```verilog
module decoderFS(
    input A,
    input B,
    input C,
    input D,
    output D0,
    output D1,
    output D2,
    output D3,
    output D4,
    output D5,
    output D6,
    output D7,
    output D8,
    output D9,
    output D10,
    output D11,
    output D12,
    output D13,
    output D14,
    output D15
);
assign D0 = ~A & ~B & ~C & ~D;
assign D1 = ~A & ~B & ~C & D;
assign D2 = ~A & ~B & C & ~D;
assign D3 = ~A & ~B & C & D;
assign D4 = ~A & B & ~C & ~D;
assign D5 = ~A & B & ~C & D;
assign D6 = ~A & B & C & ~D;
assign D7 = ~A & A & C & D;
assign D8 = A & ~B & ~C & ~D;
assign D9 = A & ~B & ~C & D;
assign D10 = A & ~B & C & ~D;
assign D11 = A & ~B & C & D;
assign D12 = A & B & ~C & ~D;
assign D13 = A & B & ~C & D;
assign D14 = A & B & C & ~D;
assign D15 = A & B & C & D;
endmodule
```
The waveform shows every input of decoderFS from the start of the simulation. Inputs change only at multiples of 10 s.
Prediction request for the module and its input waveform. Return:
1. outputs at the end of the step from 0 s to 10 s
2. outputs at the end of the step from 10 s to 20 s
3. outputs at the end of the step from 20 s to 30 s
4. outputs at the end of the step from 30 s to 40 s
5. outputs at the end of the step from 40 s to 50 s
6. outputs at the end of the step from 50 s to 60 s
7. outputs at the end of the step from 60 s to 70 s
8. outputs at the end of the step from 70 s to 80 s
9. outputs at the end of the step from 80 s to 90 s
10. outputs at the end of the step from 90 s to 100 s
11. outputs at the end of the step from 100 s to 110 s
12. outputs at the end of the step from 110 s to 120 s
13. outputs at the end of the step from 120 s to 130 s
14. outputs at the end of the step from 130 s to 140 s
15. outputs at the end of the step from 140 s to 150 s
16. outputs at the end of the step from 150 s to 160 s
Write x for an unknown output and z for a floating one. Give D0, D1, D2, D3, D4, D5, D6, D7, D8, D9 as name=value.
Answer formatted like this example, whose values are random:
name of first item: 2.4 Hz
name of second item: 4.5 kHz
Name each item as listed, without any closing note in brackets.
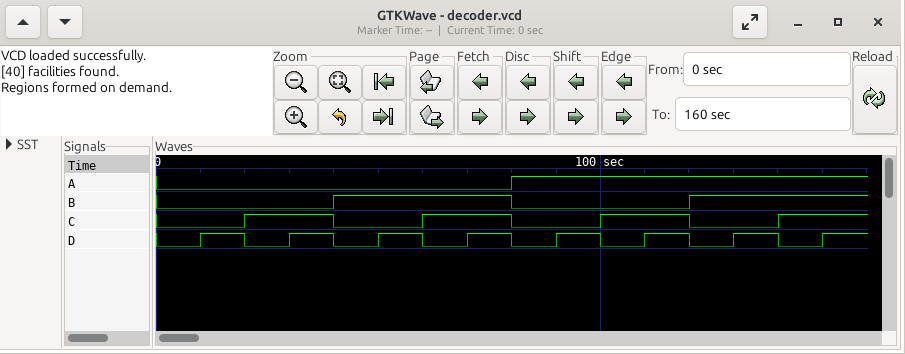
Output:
outputs at the end of the step from 0 s to 10 s: D0=1, D1=0, D2=0, D3=0, D4=0, D5=0, D6=0, D7=0, D8=0, D9=0
outputs at the end of the step from 10 s to 20 s: D0=0, D1=1, D2=0, D3=0, D4=0, D5=0, D6=0, D7=0, D8=0, D9=0
outputs at the end of the step from 20 s to 30 s: D0=0, D1=0, D2=1, D3=0, D4=0, D5=0, D6=0, D7=0, D8=0, D9=0
outputs at the end of the step from 30 s to 40 s: D0=0, D1=0, D2=0, D3=1, D4=0, D5=0, D6=0, D7=0, D8=0, D9=0
outputs at the end of the step from 40 s to 50 s: D0=0, D1=0, D2=0, D3=0, D4=1, D5=0, D6=0, D7=0, D8=0, D9=0
outputs at the end of the step from 50 s to 60 s: D0=0, D1=0, D2=0, D3=0, D4=0, D5=1, D6=0, D7=0, D8=0, D9=0
outputs at the end of the step from 60 s to 70 s: D0=0, D1=0, D2=0, D3=0, D4=0, D5=0, D6=1, D7=0, D8=0, D9=0
outputs at the end of the step from 70 s to 80 s: D0=0, D1=0, D2=0, D3=0, D4=0, D5=0, D6=0, D7=0, D8=0, D9=0
outputs at the end of the step from 80 s to 90 s: D0=0, D1=0, D2=0, D3=0, D4=0, D5=0, D6=0, D7=0, D8=1, D9=0
outputs at the end of the step from 90 s to 100 s: D0=0, D1=0, D2=0, D3=0, D4=0, D5=0, D6=0, D7=0, D8=0, D9=1
outputs at the end of the step from 100 s to 110 s: D0=0, D1=0, D2=0, D3=0, D4=0, D5=0, D6=0, D7=0, D8=0, D9=0
outputs at the end of the step from 110 s to 120 s: D0=0, D1=0, D2=0, D3=0, D4=0, D5=0, D6=0, D7=0, D8=0, D9=0
outputs at the end of the step from 120 s to 130 s: D0=0, D1=0, D2=0, D3=0, D4=0, D5=0, D6=0, D7=0, D8=0, D9=0
outputs at the end of the step from 130 s to 140 s: D0=0, D1=0, D2=0, D3=0, D4=0, D5=0, D6=0, D7=0, D8=0, D9=0
outputs at the end of the step from 140 s to 150 s: D0=0, D1=0, D2=0, D3=0, D4=0, D5=0, D6=0, D7=0, D8=0, D9=0
outputs at the end of the step from 150 s to 160 s: D0=0, D1=0, D2=0, D3=0, D4=0, D5=0, D6=0, D7=0, D8=0, D9=0
